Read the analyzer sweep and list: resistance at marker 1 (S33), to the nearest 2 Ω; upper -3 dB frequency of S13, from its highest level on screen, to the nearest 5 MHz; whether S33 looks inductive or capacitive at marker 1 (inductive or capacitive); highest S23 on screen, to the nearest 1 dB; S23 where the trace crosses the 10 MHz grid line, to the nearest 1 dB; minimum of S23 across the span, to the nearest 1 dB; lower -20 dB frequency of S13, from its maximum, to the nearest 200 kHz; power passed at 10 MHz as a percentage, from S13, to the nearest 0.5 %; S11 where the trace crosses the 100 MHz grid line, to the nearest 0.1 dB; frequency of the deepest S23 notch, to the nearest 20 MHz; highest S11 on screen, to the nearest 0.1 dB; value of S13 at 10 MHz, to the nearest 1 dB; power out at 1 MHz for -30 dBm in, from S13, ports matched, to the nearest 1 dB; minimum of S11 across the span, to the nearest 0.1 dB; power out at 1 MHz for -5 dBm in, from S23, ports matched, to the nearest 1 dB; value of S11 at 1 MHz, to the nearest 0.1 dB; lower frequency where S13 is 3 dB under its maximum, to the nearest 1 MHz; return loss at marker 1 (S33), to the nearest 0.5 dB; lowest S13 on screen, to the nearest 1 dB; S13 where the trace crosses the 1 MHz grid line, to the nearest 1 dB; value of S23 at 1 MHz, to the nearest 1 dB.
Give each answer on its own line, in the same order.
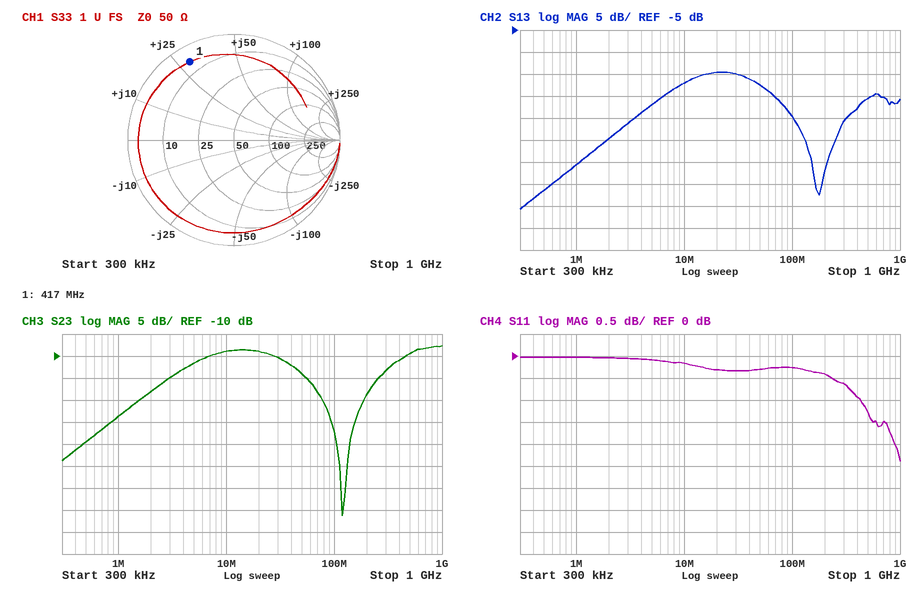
6 Ω
50 MHz
inductive
-8 dB
-9 dB
-46 dB
1.2 MHz
2.0 %
-0.3 dB
120 MHz
0.0 dB
-17 dB
-66 dBm
-2.4 dB
-29 dBm
0.0 dB
9 MHz
1.5 dB
-46 dB
-36 dB
-24 dB
